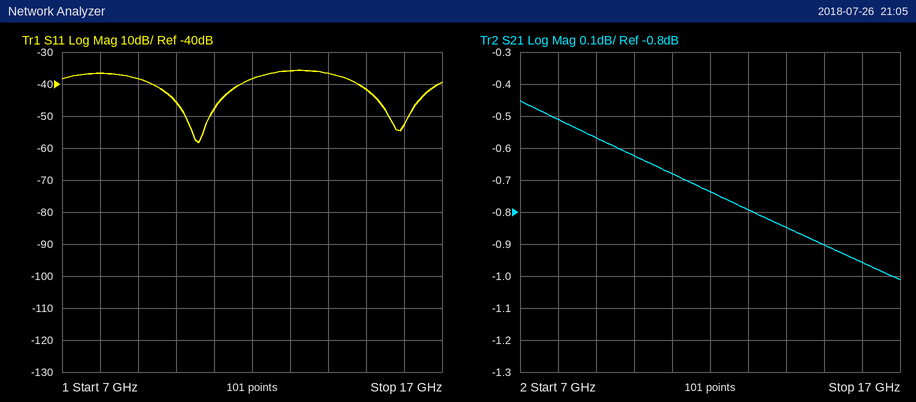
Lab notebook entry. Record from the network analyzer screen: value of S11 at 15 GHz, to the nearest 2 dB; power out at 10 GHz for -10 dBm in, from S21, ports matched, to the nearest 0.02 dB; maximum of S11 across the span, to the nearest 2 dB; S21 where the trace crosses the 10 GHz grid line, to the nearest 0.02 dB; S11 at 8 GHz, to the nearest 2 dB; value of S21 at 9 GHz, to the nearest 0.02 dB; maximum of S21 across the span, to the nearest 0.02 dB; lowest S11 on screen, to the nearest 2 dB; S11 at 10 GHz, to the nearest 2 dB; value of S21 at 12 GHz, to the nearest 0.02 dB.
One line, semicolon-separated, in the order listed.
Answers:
-42 dB; -10.62 dBm; -36 dB; -0.62 dB; -36 dB; -0.56 dB; -0.46 dB; -58 dB; -46 dB; -0.74 dB
